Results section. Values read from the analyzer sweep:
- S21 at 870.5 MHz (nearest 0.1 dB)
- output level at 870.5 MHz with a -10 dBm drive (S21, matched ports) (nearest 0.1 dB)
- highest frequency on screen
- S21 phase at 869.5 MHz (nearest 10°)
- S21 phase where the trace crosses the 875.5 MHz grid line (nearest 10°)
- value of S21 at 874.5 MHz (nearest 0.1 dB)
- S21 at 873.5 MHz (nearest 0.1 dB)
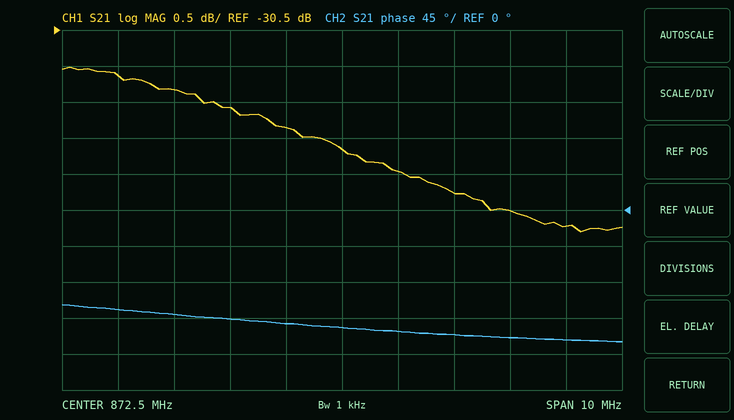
-31.6 dB
-41.6 dBm
877.5 MHz
-130°
-160°
-32.8 dB
-32.5 dB
